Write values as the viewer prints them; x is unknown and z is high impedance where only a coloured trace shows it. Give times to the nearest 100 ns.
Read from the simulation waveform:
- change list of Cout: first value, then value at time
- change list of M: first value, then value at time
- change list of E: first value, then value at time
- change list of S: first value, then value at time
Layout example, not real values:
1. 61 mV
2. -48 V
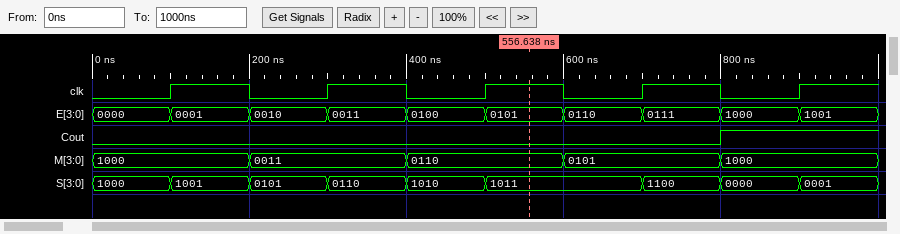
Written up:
1. 0, 1 at 800 ns
2. 1000, 0011 at 200 ns, 0110 at 400 ns, 0101 at 600 ns, 1000 at 800 ns
3. 0000, 0001 at 100 ns, 0010 at 200 ns, 0011 at 300 ns, 0100 at 400 ns, 0101 at 500 ns, 0110 at 600 ns, 0111 at 700 ns, 1000 at 800 ns, 1001 at 900 ns
4. 1000, 1001 at 100 ns, 0101 at 200 ns, 0110 at 300 ns, 1010 at 400 ns, 1011 at 500 ns, 1100 at 700 ns, 0000 at 800 ns, 0001 at 900 ns
